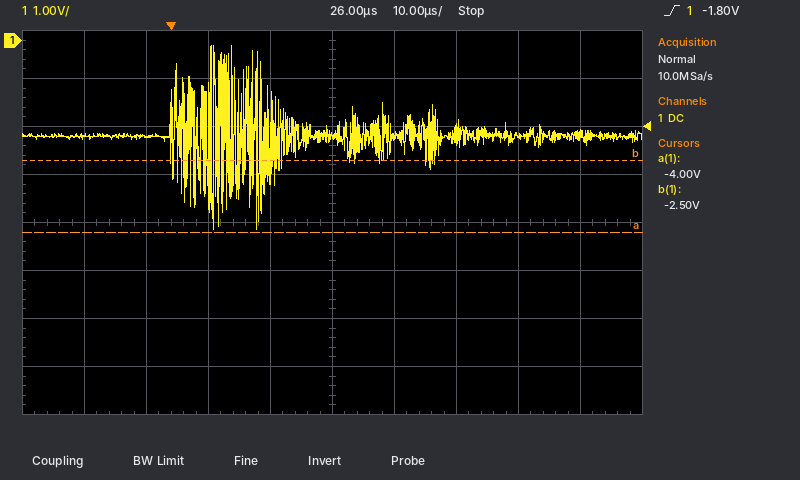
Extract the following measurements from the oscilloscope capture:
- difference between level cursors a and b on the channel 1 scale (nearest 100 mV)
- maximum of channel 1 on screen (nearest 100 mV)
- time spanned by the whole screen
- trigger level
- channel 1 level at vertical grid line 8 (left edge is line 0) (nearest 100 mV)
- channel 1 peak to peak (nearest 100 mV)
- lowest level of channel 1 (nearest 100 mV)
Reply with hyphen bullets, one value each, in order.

- 1.5 V
- -100 mV
- 100 µs
- -1.80 V
- -2.0 V
- 3.8 V
- -3.9 V
